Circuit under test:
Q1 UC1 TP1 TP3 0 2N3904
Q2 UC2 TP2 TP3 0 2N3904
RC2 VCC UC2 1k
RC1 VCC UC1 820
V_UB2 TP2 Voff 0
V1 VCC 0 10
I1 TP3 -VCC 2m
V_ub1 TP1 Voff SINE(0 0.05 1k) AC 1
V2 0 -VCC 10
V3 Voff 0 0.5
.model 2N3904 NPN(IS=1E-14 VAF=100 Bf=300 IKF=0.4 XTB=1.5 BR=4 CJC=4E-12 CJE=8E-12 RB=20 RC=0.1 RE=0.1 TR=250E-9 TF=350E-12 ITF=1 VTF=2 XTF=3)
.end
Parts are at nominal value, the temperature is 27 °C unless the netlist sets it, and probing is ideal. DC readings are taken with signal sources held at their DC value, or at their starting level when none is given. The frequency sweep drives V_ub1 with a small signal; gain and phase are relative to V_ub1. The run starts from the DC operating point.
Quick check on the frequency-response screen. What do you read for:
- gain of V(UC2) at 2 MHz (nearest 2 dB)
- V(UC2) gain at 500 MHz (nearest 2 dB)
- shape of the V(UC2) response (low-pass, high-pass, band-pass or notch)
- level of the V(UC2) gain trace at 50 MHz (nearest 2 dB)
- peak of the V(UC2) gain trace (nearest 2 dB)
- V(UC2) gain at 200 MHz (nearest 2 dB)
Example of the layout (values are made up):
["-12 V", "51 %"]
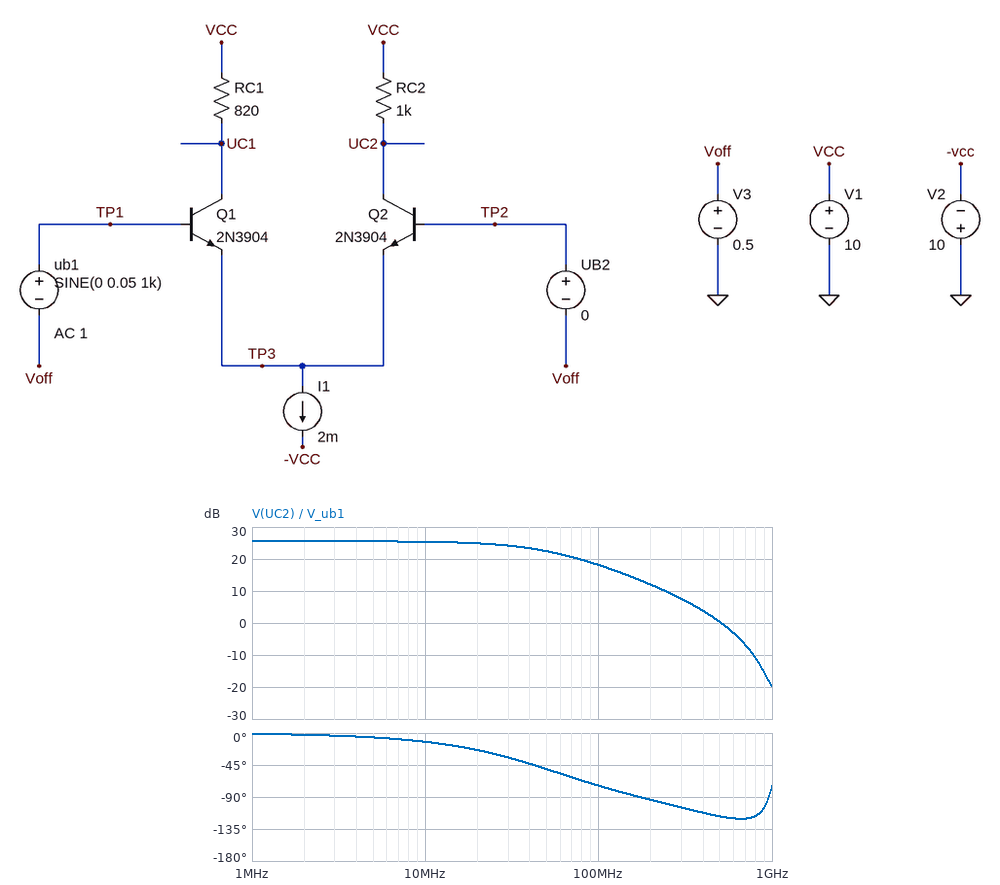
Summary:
["26 dB", "0 dB", "low-pass", "22 dB", "26 dB", "12 dB"]
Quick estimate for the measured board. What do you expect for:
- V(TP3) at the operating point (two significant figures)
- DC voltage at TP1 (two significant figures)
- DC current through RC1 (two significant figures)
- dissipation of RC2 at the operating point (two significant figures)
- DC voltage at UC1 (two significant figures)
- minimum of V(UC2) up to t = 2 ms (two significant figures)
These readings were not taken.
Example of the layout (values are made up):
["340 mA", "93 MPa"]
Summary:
["-150 mV", "500 mV", "1.0 mA", "990 µW", "9.2 V", "8.3 V"]
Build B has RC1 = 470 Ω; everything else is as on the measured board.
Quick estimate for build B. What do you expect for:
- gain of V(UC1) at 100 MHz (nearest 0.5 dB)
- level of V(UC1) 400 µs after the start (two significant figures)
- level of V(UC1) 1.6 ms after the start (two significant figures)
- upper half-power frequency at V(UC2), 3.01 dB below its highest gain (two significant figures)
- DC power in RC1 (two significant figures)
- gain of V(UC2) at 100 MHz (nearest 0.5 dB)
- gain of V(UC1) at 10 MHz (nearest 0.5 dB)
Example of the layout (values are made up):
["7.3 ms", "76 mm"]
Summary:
["15.0 dB", "9.3 V", "9.8 V", "54 MHz", "470 µW", "18.5 dB", "19.0 dB"]
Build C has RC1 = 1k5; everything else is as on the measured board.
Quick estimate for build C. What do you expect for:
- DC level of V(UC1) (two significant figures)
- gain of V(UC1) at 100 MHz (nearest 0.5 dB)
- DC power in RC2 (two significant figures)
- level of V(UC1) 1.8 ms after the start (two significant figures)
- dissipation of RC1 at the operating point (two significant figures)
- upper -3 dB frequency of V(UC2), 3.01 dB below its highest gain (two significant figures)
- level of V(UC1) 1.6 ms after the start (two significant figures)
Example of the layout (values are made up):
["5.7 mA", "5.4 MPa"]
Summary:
["8.5 V", "19.0 dB", "1.0 mW", "9.6 V", "1.5 mW", "42 MHz", "9.3 V"]
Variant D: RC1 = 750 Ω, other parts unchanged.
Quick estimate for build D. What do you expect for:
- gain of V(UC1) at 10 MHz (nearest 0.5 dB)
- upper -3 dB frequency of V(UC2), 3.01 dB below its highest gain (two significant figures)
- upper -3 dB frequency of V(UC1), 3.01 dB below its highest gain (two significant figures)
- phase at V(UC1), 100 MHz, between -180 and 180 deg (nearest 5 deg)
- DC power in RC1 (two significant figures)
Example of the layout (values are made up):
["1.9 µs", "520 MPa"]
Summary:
["23.0 dB", "50 MHz", "58 MHz", "110 deg", "750 µW"]
